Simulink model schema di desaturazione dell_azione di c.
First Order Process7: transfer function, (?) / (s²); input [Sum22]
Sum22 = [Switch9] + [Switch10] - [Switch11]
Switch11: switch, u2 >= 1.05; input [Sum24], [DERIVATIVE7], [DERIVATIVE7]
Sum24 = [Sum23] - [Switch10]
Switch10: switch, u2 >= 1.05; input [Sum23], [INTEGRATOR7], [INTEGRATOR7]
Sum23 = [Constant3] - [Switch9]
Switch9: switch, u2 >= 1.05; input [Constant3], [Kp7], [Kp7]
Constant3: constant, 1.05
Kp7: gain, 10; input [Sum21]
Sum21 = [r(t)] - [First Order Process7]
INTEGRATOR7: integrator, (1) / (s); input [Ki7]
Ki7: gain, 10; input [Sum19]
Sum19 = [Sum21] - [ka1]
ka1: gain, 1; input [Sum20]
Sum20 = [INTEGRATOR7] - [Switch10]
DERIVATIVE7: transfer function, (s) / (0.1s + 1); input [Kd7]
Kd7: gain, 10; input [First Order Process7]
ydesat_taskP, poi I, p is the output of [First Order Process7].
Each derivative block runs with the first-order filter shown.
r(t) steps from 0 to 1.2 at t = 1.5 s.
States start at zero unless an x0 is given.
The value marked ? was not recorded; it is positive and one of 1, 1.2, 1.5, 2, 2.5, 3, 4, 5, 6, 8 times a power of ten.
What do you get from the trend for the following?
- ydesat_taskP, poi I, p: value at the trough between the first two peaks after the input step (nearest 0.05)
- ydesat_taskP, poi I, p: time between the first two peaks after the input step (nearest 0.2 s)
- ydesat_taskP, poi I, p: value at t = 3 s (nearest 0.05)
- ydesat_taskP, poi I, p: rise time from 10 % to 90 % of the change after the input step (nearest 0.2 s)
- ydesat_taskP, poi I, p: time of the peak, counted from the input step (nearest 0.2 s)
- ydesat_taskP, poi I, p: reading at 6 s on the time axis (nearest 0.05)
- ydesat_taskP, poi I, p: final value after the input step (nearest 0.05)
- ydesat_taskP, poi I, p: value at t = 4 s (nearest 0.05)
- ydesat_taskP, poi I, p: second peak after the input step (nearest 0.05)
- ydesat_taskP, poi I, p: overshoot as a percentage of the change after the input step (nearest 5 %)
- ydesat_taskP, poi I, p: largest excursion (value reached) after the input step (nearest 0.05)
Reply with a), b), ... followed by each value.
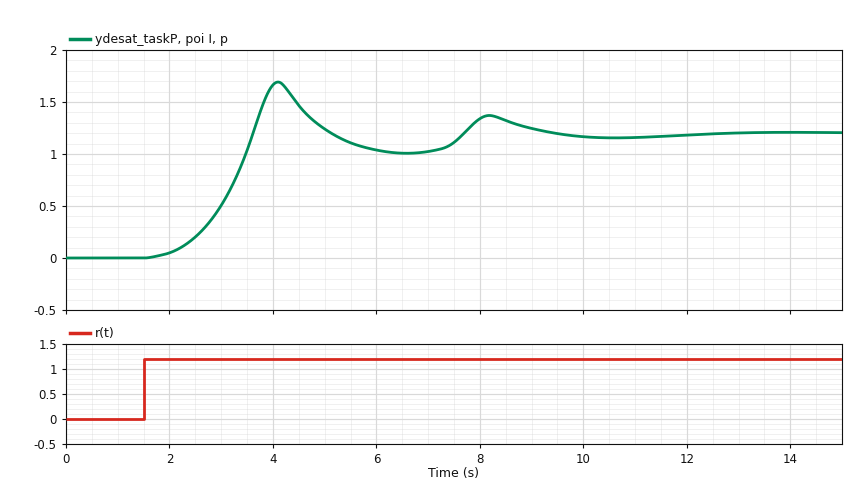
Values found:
a) 1.00
b) 4.0 s
c) 0.50
d) 1.2 s
e) 2.6 s
f) 1.05
g) 1.20
h) 1.65
i) 1.35
j) 40 %
k) 1.70
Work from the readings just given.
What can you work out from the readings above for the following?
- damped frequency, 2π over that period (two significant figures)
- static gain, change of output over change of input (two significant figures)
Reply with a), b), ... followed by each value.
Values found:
a) 1.6 rad/s
b) 1.0
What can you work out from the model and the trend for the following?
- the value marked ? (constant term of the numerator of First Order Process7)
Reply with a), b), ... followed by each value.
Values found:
a) 0.5
